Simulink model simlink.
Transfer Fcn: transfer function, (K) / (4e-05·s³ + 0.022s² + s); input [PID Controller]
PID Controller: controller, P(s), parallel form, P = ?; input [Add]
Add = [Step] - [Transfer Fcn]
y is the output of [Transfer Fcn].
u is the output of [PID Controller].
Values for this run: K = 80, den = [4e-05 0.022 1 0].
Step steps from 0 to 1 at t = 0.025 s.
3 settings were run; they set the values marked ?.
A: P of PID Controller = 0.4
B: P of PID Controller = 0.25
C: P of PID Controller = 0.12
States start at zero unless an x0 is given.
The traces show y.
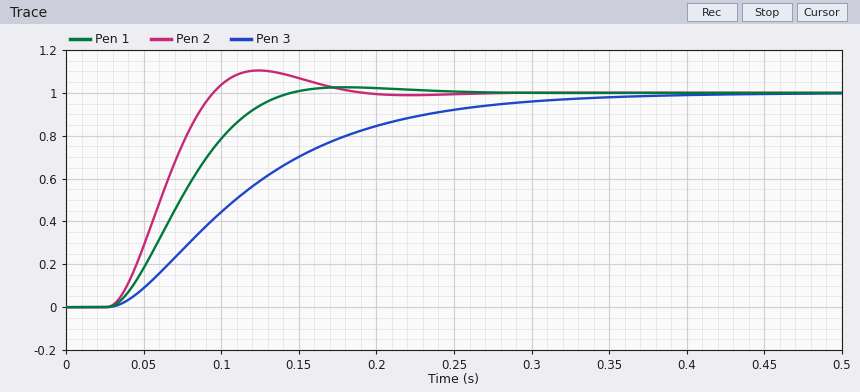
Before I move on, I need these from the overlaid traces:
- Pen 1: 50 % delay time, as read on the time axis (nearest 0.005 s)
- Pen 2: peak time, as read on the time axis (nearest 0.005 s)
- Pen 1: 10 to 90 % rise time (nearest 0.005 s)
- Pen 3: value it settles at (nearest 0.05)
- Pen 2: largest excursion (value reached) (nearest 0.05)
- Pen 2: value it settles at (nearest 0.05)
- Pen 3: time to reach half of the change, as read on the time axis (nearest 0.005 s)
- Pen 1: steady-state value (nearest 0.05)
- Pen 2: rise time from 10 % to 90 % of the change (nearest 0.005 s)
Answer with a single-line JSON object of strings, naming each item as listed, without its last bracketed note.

{"Pen 1: 50 % delay time, as read on the time axis": "0.075 s", "Pen 2: peak time, as read on the time axis": "0.125 s", "Pen 1: 10 to 90 % rise time": "0.075 s", "Pen 3: value it settles at": "1.00", "Pen 2: largest excursion (value reached)": "1.10", "Pen 2: value it settles at": "1.00", "Pen 3: time to reach half of the change, as read on the time axis": "0.110 s", "Pen 1: steady-state value": "1.00", "Pen 2: rise time from 10 % to 90 % of the change": "0.045 s"}
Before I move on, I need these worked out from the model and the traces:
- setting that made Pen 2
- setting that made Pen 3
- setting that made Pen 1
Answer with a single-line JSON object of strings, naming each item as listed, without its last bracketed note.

{"setting that made Pen 2": "A", "setting that made Pen 3": "C", "setting that made Pen 1": "B"}
